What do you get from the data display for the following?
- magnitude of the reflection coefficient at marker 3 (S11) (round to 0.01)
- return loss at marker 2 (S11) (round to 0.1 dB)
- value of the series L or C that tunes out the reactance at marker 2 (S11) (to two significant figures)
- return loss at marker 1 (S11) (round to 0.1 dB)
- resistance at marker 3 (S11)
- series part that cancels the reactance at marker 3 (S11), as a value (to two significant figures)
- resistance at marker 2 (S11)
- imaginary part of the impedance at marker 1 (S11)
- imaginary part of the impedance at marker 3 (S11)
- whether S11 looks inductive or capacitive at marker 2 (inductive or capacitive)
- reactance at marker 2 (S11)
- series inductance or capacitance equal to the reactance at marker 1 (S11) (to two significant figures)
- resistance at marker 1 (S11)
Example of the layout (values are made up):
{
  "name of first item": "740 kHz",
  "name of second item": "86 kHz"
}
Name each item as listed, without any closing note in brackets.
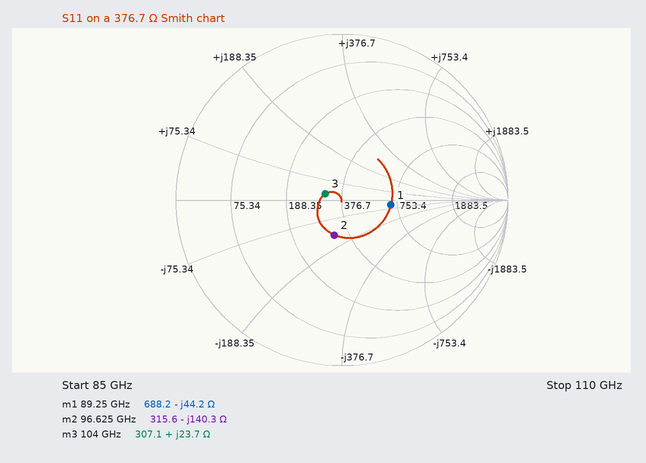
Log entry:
{
  "magnitude of the reflection coefficient at marker 3 (S11)": "0.11",
  "return loss at marker 2 (S11)": "13.3 dB",
  "value of the series L or C that tunes out the reactance at marker 2 (S11)": "230 pH",
  "return loss at marker 1 (S11)": "10.6 dB",
  "resistance at marker 3": "307.1 Ω",
  "series part that cancels the reactance at marker 3 (S11), as a value": "65 fF",
  "resistance at marker 2": "315.6 Ω",
  "imaginary part of the impedance at marker 1": "-44.2 Ω",
  "imaginary part of the impedance at marker 3": "+23.7 Ω",
  "whether S11 looks inductive or capacitive at marker 2": "capacitive",
  "reactance at marker 2": "-140.3 Ω",
  "series inductance or capacitance equal to the reactance at marker 1 (S11)": "40 fF",
  "resistance at marker 1": "688.2 Ω"
}
